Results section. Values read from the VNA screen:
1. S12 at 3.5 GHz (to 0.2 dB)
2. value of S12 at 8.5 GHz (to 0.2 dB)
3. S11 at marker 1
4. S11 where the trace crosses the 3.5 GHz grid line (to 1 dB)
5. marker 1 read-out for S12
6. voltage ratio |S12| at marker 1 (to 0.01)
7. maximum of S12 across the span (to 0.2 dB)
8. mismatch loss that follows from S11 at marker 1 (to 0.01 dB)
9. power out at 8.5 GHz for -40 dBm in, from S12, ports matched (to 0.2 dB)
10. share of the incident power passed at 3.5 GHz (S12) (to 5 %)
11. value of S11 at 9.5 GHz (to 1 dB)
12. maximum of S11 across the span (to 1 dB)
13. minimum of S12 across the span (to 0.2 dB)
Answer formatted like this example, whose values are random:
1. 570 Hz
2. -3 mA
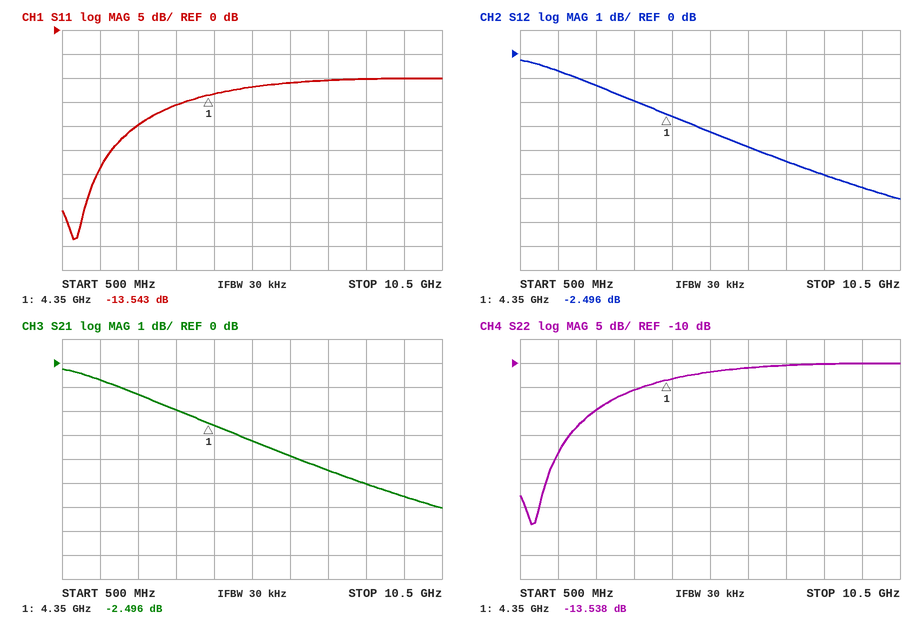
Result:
1. -2.0 dB
2. -5.0 dB
3. -13.543 dB
4. -16 dB
5. -2.496 dB
6. 0.75
7. -0.2 dB
8. 0.20 dB
9. -45.0 dBm
10. 65 %
11. -10 dB
12. -10 dB
13. -6.0 dB
